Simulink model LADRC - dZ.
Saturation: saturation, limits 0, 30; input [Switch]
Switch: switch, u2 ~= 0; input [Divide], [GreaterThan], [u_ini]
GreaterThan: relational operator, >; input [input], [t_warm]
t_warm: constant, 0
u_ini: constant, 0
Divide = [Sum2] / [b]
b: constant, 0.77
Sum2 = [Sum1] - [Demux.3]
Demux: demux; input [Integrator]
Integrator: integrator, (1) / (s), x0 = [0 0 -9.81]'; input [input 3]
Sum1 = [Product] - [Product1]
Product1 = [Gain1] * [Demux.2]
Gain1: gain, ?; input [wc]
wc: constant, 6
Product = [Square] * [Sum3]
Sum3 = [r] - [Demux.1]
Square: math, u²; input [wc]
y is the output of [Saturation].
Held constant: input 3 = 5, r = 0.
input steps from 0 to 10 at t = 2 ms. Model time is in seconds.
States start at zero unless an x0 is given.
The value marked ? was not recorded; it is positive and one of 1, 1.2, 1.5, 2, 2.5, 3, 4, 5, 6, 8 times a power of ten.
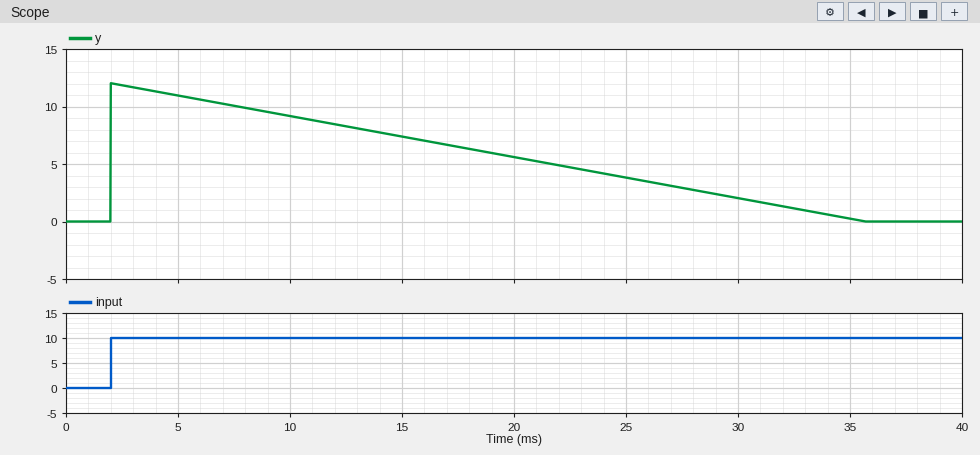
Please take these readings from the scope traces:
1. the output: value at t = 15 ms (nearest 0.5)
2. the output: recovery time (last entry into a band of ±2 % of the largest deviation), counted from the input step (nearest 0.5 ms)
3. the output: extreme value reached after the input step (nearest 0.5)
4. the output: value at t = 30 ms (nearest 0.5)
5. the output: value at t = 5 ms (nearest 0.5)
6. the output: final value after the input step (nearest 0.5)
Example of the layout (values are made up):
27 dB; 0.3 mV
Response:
7.5; 33.0 ms; 12.0; 2.0; 11.0; 0.0
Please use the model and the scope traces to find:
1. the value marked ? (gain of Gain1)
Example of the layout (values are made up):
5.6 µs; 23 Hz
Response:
3
